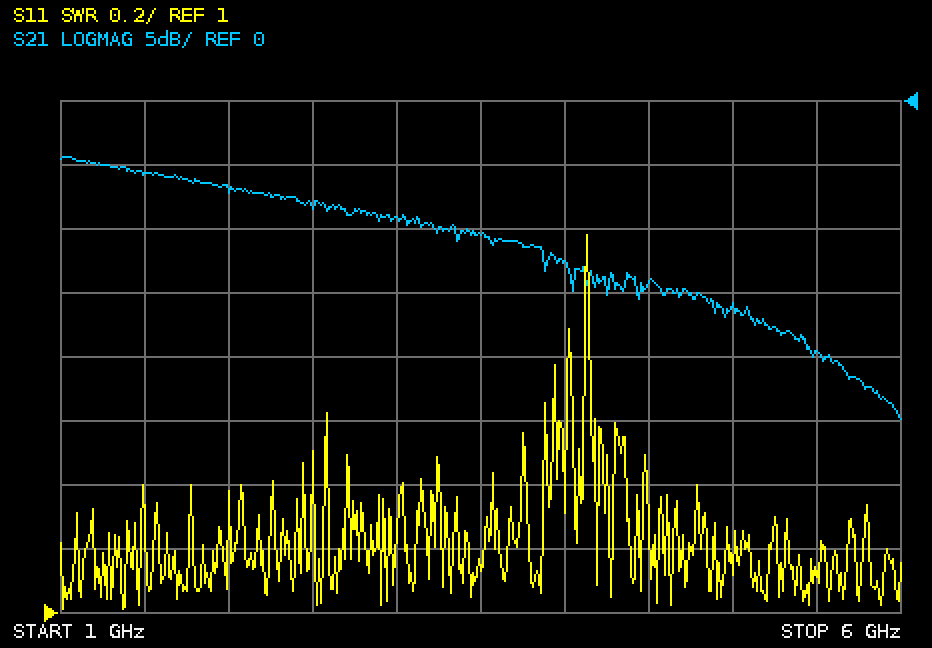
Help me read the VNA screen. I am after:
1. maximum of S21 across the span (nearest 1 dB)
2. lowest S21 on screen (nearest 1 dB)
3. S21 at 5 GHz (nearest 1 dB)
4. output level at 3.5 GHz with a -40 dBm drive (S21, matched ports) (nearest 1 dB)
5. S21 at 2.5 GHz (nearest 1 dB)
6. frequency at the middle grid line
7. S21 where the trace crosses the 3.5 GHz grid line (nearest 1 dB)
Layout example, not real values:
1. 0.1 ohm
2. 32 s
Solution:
1. -4 dB
2. -25 dB
3. -16 dB
4. -50 dBm
5. -8 dB
6. 3.5 GHz
7. -10 dB
